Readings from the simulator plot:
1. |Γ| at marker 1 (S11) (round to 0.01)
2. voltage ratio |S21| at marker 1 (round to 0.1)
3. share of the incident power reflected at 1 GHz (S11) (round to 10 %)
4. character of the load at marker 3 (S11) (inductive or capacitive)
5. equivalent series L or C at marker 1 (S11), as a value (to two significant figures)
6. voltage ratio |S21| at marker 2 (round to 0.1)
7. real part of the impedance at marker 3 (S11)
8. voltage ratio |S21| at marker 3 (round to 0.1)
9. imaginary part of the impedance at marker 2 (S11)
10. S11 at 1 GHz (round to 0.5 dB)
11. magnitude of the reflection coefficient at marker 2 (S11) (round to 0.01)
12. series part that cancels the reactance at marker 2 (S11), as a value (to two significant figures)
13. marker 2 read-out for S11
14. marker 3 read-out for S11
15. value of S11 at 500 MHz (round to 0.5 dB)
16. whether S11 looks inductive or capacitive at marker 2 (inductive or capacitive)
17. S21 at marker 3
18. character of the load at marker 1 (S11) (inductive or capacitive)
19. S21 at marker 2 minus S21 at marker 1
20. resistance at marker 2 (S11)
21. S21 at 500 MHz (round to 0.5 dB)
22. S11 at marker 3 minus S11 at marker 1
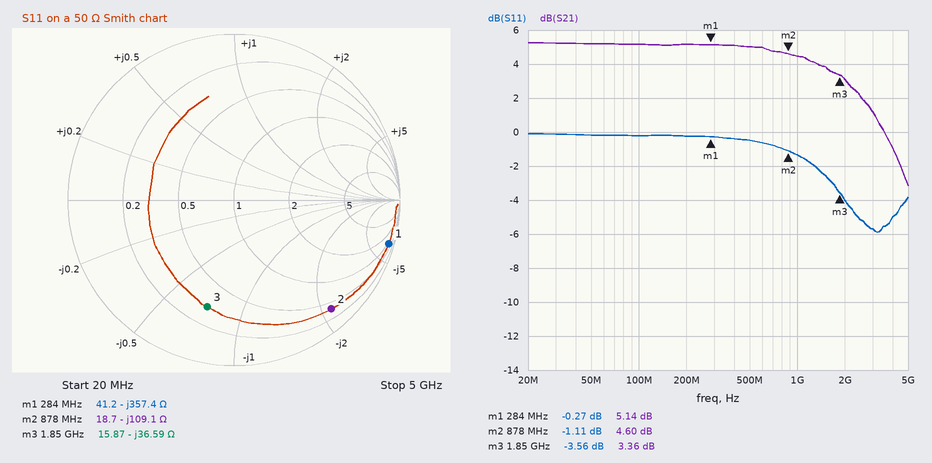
0.97
1.8
70 %
capacitive
1.6 pF
1.7
15.87 Ω
1.5
-109.1 Ω
-1.5 dB
0.88
20 nH
-1.11 dB
-3.56 dB
-0.5 dB
capacitive
3.36 dB
capacitive
-0.54 dB
18.7 Ω
5.0 dB
-3.29 dB
